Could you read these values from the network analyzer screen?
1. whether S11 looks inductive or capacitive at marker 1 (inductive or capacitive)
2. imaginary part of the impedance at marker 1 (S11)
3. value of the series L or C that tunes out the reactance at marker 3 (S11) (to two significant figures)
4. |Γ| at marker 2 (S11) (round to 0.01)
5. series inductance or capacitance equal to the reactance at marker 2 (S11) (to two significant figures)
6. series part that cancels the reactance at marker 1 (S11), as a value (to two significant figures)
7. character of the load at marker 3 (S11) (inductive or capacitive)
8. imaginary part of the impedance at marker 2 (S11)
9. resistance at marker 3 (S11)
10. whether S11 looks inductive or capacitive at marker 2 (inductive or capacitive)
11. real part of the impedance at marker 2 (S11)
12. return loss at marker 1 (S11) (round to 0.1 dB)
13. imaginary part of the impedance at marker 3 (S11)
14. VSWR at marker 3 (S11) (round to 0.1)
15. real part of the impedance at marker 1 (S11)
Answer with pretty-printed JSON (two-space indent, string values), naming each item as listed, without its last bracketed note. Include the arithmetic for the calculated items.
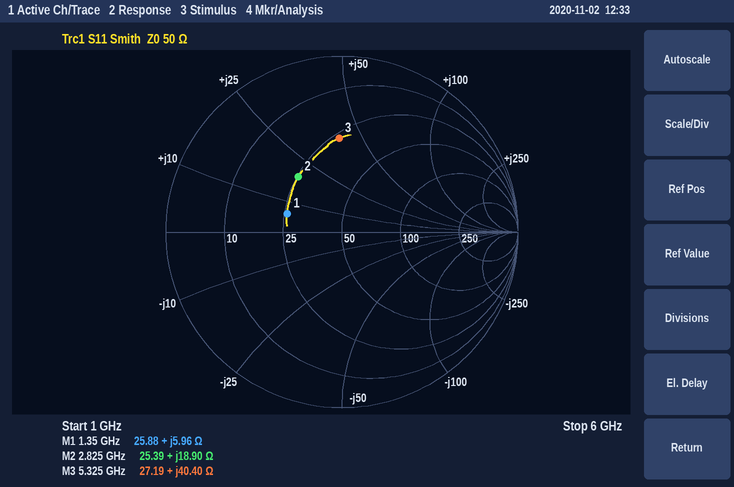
{
  "whether S11 looks inductive or capacitive at marker 1": "inductive",
  "imaginary part of the impedance at marker 1": "+5.96 Ω",
  "value of the series L or C that tunes out the reactance at marker 3 (S11)": "C = 1/(2π × 5.325 GHz × 40.4 Ω) ≈ 740 fF",
  "|Γ| at marker 2 (S11)": "0.40",
  "series inductance or capacitance equal to the reactance at marker 2 (S11)": "L = 18.9 Ω/(2π × 2.825 GHz) ≈ 1.1 nH",
  "series part that cancels the reactance at marker 1 (S11), as a value": "C = 1/(2π × 1.35 GHz × 5.96 Ω) ≈ 20 pF",
  "character of the load at marker 3 (S11)": "inductive",
  "imaginary part of the impedance at marker 2": "+18.90 Ω",
  "resistance at marker 3": "27.19 Ω",
  "whether S11 looks inductive or capacitive at marker 2": "inductive",
  "real part of the impedance at marker 2": "25.39 Ω",
  "return loss at marker 1 (S11)": "9.7 dB",
  "imaginary part of the impedance at marker 3": "+40.40 Ω",
  "VSWR at marker 3 (S11)": "3.3",
  "real part of the impedance at marker 1": "25.88 Ω"
}
